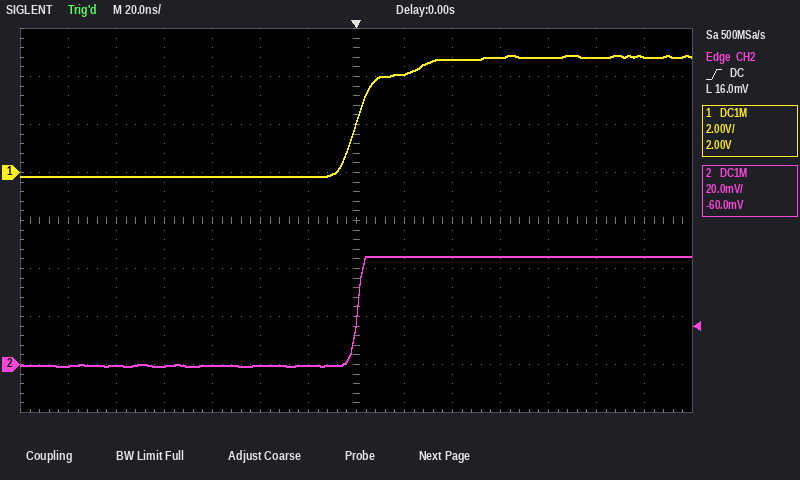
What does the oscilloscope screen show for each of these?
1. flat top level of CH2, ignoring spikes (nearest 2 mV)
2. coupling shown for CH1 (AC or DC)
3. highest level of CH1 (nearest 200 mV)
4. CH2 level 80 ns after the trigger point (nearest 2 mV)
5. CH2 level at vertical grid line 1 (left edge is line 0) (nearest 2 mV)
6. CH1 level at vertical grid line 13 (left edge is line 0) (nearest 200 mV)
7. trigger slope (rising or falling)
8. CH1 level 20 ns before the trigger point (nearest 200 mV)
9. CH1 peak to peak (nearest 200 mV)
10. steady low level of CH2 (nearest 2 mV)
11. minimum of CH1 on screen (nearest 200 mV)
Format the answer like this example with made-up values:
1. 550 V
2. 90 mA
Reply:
1. 44 mV
2. DC
3. 4.8 V
4. 44 mV
5. 0 mV
6. 4.8 V
7. rising
8. -200 mV
9. 5.0 V
10. 0 mV
11. -200 mV
